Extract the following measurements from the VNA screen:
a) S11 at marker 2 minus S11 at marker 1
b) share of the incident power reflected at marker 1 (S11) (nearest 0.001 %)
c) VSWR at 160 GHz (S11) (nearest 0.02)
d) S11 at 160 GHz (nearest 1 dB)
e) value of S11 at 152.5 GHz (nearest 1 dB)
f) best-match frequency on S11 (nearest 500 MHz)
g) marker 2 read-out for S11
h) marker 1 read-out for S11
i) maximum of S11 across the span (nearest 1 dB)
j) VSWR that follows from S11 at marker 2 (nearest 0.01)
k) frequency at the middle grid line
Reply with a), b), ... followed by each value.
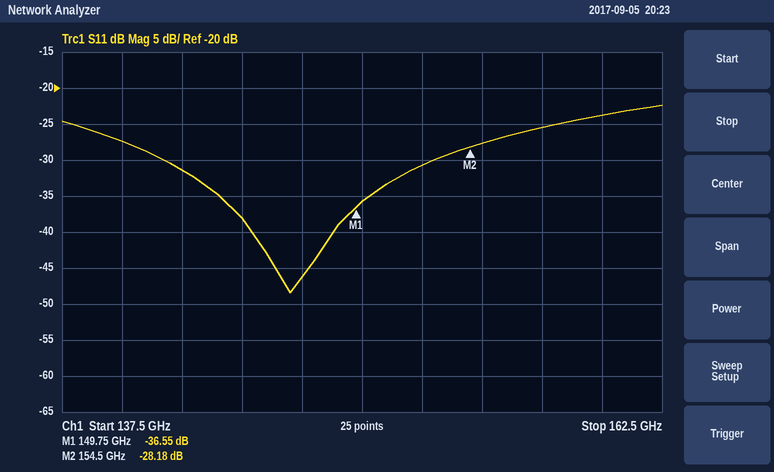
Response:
a) 8.37 dB
b) 0.022 %
c) 1.14
d) -24 dB
e) -31 dB
f) 147.0 GHz
g) -28.18 dB
h) -36.55 dB
i) -22 dB
j) 1.08
k) 150 GHz
